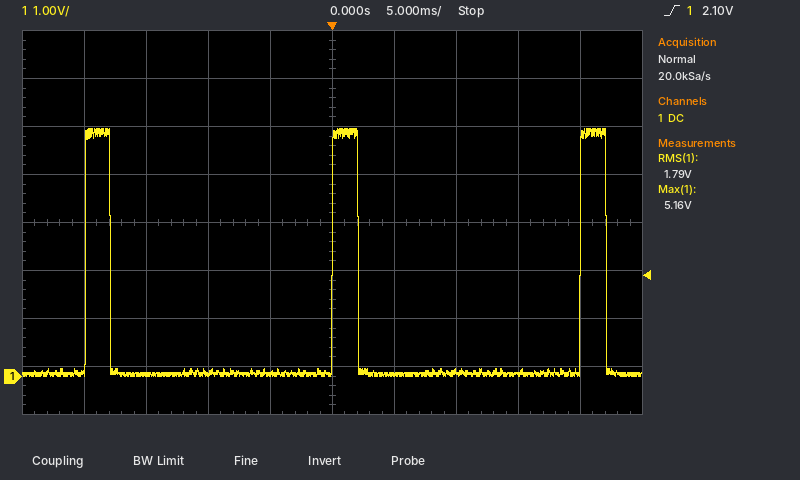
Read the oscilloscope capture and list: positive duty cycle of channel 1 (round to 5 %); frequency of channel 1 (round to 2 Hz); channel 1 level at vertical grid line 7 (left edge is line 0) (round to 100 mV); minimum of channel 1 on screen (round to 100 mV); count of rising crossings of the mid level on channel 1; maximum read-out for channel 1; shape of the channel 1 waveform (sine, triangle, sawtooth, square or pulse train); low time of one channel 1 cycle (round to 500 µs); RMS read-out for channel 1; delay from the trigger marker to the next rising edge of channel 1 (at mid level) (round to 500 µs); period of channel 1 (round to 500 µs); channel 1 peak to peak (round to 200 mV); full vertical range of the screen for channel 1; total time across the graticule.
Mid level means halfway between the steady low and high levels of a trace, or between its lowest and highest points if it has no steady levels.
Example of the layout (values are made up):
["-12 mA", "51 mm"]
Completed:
["10 %", "50 Hz", "100 mV", "0.0 V", "3", "5.16 V", "pulse train", "18.0 ms", "1.79 V", "20.0 ms", "20.0 ms", "5.2 V", "8 V", "50 ms"]
